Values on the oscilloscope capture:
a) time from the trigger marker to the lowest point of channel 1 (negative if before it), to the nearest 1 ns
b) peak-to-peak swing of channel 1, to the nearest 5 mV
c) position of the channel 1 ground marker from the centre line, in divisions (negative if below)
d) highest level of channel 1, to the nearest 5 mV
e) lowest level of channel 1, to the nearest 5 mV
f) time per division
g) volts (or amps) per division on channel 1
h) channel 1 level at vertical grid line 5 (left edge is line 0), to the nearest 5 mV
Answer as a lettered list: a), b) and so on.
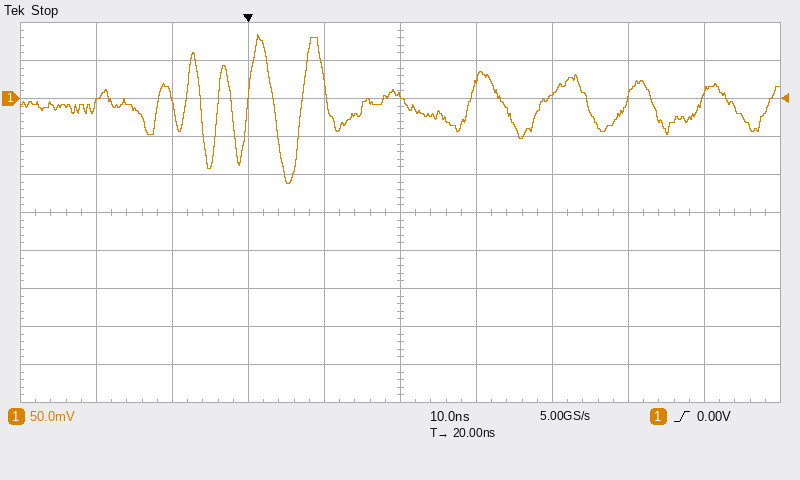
a) +5 ns
b) 195 mV
c) +3.0 div
d) 85 mV
e) -110 mV
f) 10 ns
g) 50 mV
h) 5 mV
